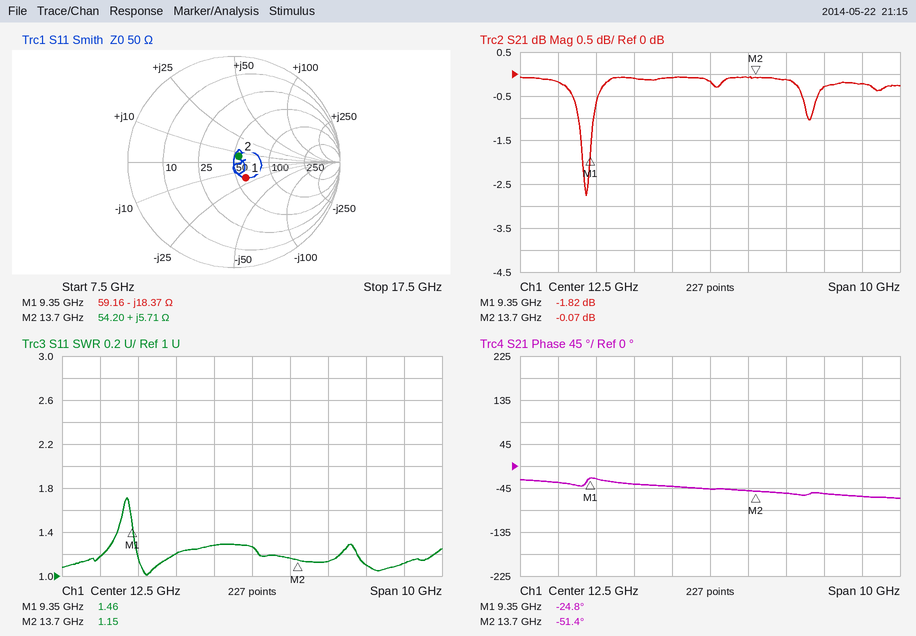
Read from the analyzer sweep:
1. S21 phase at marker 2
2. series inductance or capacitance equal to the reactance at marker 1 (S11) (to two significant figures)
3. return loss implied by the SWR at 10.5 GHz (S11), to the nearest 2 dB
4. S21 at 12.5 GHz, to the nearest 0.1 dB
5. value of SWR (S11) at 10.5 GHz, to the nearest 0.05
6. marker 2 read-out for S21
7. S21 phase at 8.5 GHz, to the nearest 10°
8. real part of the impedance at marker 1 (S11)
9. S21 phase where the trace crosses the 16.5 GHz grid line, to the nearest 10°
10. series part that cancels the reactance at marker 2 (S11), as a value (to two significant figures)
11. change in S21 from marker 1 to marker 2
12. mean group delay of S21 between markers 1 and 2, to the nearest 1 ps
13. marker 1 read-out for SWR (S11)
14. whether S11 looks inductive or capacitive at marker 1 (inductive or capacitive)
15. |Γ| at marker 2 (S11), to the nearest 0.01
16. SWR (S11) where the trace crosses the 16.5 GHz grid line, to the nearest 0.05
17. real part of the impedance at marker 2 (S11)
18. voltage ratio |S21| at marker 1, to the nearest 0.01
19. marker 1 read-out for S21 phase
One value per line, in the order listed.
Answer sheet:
-51.4°
930 fF
20 dB
-0.2 dB
1.20
-0.07 dB
-30°
59.16 Ω
-60°
2.0 pF
1.75 dB
17 ps
1.46
capacitive
0.07
1.10
54.20 Ω
0.81
-24.8°
